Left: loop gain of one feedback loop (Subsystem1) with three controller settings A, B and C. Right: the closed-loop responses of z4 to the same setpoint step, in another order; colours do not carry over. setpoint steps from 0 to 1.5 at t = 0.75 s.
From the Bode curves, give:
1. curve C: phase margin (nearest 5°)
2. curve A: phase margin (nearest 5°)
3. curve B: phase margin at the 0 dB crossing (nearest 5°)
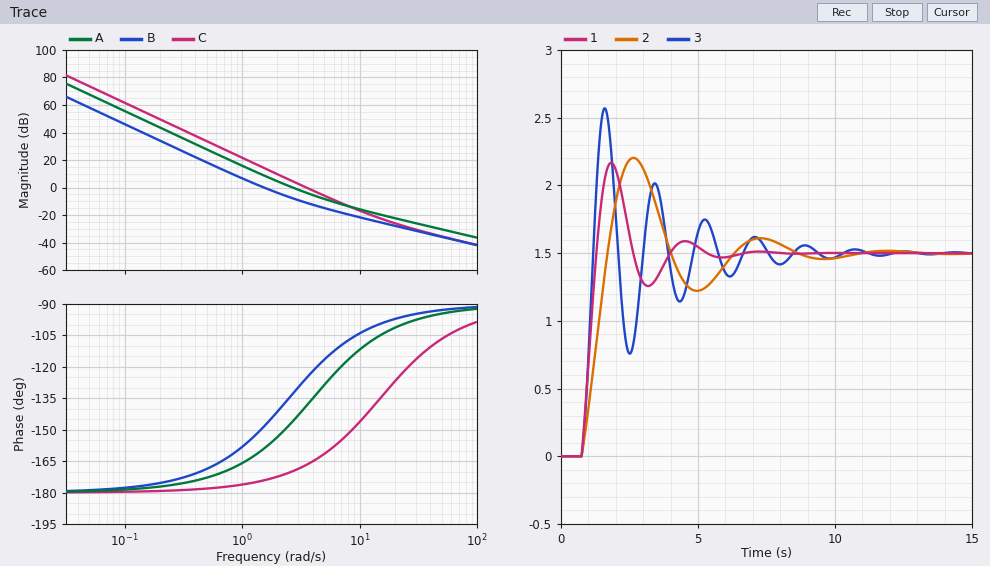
15°
35°
30°
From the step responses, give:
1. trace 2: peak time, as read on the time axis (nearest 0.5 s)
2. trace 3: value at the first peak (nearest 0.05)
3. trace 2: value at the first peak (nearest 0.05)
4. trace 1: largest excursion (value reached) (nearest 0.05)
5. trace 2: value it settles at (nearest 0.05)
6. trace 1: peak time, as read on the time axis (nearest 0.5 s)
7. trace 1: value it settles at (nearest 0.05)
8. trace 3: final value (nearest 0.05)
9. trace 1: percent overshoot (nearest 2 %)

2.5 s
2.55
2.20
2.15
1.50
2.0 s
1.50
1.50
44 %
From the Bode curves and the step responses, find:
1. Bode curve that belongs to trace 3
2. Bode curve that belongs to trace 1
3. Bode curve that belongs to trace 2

C
A
B
